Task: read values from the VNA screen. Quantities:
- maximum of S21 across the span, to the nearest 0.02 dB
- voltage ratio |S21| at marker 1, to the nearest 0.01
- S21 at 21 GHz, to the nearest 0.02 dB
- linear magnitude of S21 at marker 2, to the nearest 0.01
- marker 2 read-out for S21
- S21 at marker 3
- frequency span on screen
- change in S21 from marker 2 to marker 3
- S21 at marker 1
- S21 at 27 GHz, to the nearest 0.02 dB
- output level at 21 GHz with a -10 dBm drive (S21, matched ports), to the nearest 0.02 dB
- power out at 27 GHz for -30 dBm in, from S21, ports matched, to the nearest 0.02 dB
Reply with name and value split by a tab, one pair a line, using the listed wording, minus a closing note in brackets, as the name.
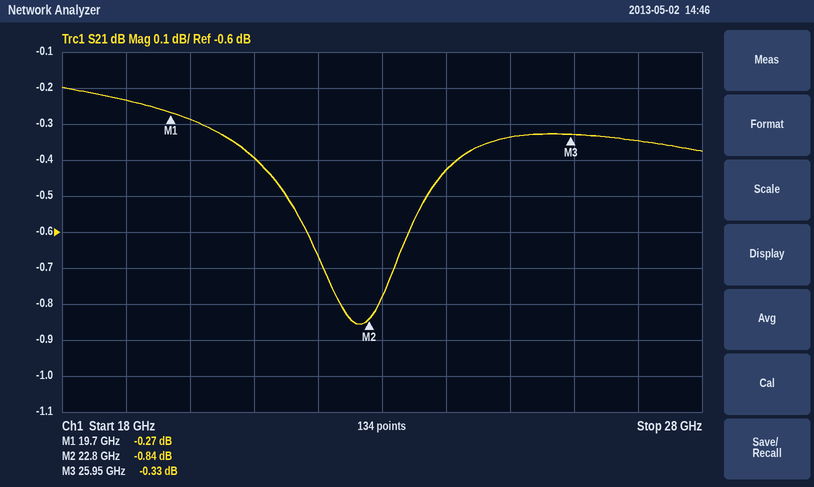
maximum of S21 across the span, to the nearest 0.02 dB	-0.20 dB
voltage ratio |S21| at marker 1, to the nearest 0.01	0.97
S21 at 21 GHz, to the nearest 0.02 dB	-0.40 dB
linear magnitude of S21 at marker 2, to the nearest 0.01	0.91
marker 2 read-out for S21	-0.84 dB
S21 at marker 3	-0.33 dB
frequency span on screen	10 GHz
change in S21 from marker 2 to marker 3	0.51 dB
S21 at marker 1	-0.27 dB
S21 at 27 GHz, to the nearest 0.02 dB	-0.34 dB
output level at 21 GHz with a -10 dBm drive (S21, matched ports), to the nearest 0.02 dB	-10.40 dBm
power out at 27 GHz for -30 dBm in, from S21, ports matched, to the nearest 0.02 dB	-30.34 dBm
